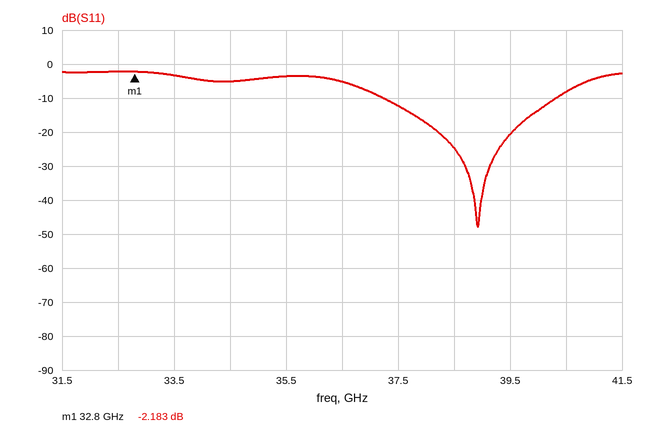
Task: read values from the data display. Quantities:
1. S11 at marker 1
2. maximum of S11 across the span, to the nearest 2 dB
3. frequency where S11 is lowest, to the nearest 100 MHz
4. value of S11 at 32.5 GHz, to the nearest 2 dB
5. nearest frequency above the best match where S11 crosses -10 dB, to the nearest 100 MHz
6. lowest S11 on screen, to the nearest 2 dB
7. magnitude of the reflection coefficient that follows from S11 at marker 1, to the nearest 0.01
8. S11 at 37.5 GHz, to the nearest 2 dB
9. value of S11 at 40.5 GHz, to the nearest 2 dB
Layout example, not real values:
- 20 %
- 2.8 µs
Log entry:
- -2.183 dB
- -2 dB
- 38.9 GHz
- -2 dB
- 40.3 GHz
- -48 dB
- 0.78
- -12 dB
- -8 dB
